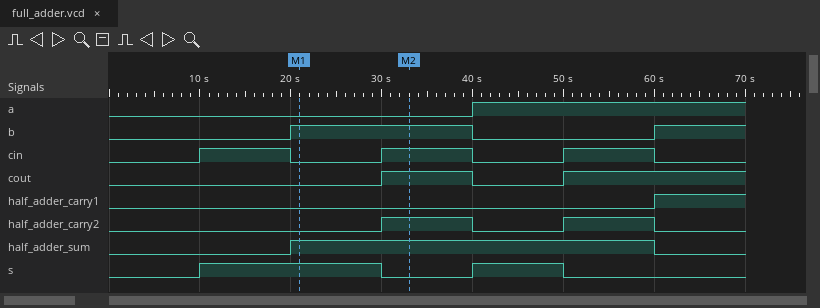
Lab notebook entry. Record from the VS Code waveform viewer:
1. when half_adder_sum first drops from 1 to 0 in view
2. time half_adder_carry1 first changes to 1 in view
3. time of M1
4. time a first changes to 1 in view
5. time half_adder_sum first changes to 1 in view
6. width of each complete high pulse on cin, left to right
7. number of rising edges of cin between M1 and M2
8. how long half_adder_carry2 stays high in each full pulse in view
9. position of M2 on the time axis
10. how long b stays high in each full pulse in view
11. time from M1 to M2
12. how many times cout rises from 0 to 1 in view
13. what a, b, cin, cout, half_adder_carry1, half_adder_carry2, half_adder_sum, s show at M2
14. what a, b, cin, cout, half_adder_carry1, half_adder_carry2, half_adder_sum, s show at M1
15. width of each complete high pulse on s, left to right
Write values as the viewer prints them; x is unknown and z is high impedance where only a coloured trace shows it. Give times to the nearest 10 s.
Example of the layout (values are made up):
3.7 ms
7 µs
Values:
60 s
60 s
20 s
40 s
20 s
10 s, 10 s, 10 s
1
10 s, 10 s
30 s
20 s
10 s
2
a=0, b=1, cin=1, cout=1, half_adder_carry1=0, half_adder_carry2=1, half_adder_sum=1, s=0
a=0, b=1, cin=0, cout=0, half_adder_carry1=0, half_adder_carry2=0, half_adder_sum=1, s=1
20 s, 10 s
